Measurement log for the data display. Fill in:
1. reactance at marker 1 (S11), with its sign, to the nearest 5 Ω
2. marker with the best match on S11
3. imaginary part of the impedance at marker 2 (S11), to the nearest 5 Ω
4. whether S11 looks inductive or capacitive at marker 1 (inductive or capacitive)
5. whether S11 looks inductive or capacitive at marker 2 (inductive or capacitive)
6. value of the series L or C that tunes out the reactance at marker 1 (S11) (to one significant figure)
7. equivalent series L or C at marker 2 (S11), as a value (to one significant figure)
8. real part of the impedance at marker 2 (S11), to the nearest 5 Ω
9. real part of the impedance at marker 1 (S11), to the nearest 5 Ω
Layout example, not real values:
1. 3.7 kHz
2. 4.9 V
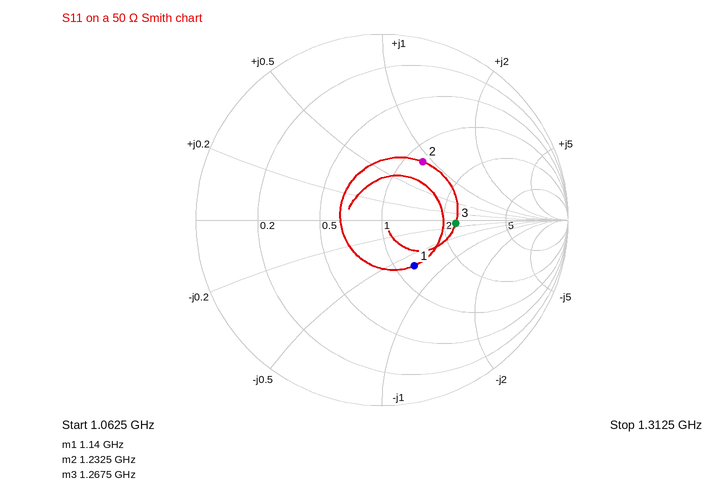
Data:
1. -35 Ω
2. marker 1
3. +45 Ω
4. capacitive
5. inductive
6. 5 nH
7. 6 nH
8. 60 Ω
9. 60 Ω
